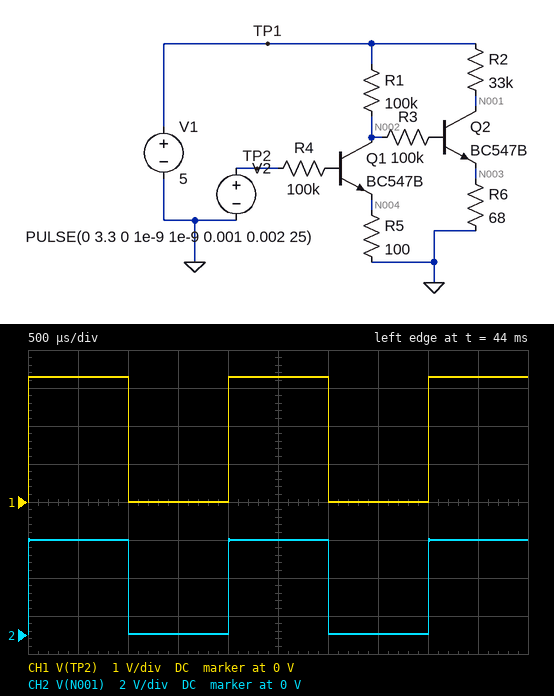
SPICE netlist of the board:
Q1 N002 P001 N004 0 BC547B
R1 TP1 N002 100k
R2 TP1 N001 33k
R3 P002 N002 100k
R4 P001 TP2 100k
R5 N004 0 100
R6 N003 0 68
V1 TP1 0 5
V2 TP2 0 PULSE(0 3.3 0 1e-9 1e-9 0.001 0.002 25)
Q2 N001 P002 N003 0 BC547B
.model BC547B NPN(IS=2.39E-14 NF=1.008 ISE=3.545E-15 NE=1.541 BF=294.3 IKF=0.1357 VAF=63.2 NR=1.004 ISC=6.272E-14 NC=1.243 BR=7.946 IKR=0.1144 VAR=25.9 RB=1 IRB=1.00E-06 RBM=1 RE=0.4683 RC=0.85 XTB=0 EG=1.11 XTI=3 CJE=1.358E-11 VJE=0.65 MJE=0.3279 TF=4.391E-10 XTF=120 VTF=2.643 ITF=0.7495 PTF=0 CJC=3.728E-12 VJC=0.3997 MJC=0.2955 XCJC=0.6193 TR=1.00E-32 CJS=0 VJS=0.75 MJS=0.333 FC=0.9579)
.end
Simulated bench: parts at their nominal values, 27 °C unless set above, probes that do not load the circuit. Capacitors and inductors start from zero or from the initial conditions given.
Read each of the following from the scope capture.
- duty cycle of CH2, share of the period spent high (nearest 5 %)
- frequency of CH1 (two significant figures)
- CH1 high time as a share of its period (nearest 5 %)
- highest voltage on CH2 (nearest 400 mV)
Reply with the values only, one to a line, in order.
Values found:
50 %
500 Hz
50 %
5.2 V
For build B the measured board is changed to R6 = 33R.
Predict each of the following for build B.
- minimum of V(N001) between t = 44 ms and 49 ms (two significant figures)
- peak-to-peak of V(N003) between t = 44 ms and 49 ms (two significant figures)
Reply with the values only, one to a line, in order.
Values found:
30 mV
5.9 mV
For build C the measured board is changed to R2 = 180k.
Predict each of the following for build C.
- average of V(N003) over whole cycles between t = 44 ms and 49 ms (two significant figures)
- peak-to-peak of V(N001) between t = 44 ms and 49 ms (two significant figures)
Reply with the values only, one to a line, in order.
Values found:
1.7 mV
5.1 V
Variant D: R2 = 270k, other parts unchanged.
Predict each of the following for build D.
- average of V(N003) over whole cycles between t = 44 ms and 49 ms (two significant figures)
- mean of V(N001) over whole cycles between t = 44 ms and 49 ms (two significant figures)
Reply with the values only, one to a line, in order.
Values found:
1.4 mV
2.5 V
